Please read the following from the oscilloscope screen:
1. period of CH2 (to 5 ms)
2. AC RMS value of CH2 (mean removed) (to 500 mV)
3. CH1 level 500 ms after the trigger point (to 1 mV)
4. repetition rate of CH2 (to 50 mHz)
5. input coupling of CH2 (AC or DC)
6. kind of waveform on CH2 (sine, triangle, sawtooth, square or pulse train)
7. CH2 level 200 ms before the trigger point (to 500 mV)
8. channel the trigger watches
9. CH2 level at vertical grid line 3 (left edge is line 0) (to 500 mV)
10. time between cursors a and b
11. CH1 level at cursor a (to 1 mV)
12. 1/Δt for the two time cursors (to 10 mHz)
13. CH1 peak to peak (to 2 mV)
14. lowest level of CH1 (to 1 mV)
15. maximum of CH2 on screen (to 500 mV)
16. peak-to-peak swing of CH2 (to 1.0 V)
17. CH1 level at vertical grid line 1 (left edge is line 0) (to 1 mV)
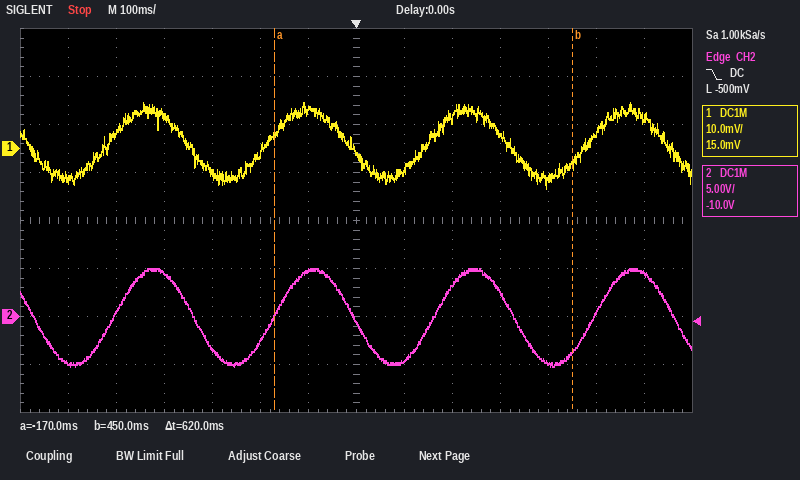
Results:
335 ms
3.5 V
3 mV
3.00 Hz
DC
sine
-2.5 V
CH2
4.5 V
620 ms
3 mV
1.61 Hz
18 mV
-8 mV
5.0 V
10.0 V
-6 mV
